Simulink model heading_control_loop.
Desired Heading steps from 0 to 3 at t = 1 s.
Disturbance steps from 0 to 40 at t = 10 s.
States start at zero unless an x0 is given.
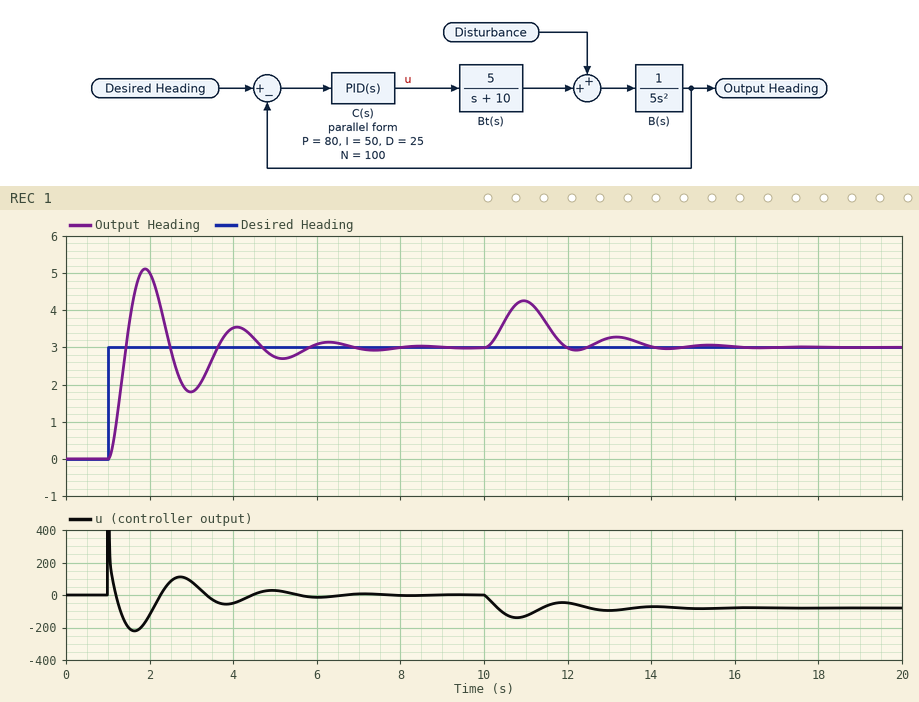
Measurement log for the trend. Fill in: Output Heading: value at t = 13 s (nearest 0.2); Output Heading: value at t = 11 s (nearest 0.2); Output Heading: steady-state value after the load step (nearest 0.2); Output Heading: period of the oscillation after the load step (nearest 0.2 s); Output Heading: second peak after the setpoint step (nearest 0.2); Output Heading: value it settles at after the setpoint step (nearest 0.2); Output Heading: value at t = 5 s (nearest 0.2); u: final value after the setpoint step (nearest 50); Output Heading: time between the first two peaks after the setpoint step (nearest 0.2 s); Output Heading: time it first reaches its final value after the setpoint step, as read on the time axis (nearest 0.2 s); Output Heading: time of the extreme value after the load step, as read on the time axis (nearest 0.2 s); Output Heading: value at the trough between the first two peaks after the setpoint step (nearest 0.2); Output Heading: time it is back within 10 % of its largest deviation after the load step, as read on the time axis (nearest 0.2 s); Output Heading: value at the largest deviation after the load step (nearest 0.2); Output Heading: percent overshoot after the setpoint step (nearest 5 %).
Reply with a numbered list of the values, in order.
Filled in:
1. 3.2
2. 4.2
3. 3.0
4. 2.2 s
5. 3.6
6. 3.0
7. 2.8
8. 0
9. 2.2 s
10. 1.4 s
11. 11.0 s
12. 1.8
13. 13.8 s
14. 4.2
15. 70 %
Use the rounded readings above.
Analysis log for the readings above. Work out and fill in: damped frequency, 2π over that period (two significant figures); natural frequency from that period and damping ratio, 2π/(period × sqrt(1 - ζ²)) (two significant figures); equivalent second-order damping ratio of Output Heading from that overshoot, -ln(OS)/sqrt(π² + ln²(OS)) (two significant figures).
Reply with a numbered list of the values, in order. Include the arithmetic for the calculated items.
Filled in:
1. 2π / 2.2 = 2.9 rad/s
2. 2π / (2.2 × sqrt(1 - 0.11²)) = 2.9 rad/s
3. ln(0.7) = -0.357; 0.357 / sqrt(9.870 + 0.127) = 0.11
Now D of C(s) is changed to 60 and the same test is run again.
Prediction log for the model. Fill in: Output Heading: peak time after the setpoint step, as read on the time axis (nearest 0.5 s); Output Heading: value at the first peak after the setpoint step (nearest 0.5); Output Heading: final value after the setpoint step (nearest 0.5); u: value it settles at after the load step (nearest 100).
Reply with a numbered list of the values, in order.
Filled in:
1. 1.5 s
2. 4.0
3. 3.0
4. -100
